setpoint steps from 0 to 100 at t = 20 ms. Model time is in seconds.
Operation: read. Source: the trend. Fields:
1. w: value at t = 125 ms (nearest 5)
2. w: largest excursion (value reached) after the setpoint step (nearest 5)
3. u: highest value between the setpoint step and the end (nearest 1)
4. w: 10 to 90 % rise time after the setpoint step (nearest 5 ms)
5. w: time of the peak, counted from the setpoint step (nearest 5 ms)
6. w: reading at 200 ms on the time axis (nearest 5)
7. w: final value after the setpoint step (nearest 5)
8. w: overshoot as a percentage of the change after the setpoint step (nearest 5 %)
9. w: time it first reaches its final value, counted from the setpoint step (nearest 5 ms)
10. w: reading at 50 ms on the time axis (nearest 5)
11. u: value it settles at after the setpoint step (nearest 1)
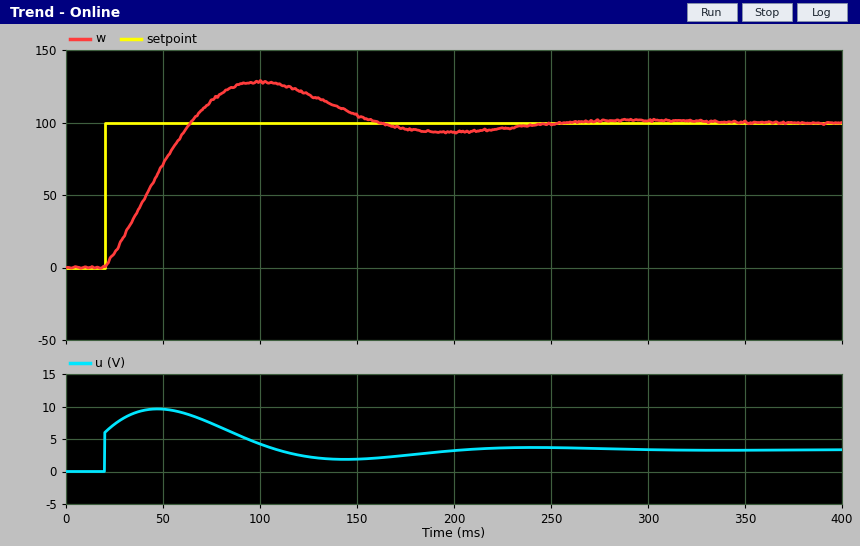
120
130
10
35 ms
80 ms
95
100
30 %
45 ms
70
3
